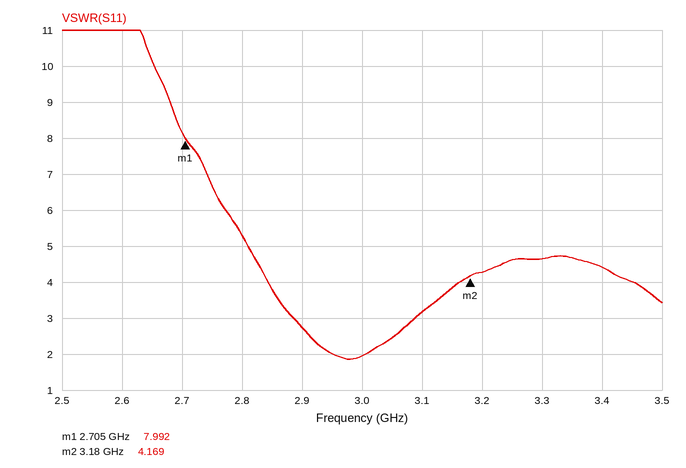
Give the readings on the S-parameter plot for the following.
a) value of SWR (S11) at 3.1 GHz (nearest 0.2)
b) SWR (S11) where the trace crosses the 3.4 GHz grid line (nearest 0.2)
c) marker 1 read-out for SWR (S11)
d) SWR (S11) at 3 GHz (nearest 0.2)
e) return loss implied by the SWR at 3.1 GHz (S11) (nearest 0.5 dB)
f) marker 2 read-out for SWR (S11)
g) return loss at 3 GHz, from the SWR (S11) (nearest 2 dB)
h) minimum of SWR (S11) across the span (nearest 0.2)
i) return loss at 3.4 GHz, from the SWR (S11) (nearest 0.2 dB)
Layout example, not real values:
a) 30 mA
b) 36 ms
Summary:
a) 3.2
b) 4.4
c) 7.992
d) 2.0
e) 5.5 dB
f) 4.169
g) 10 dB
h) 1.8
i) 4.0 dB
